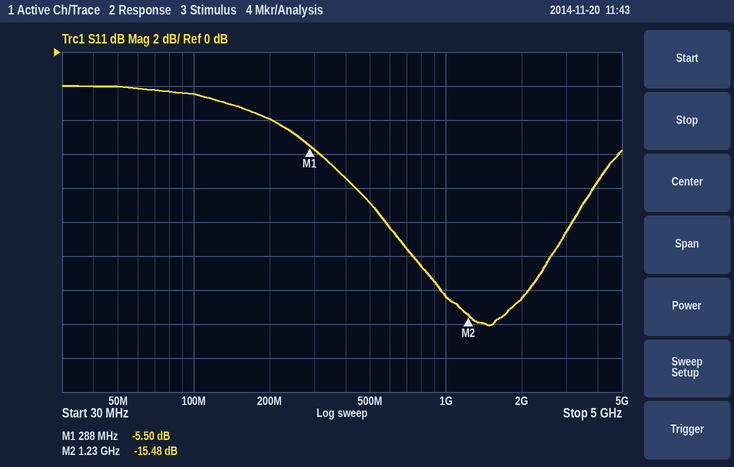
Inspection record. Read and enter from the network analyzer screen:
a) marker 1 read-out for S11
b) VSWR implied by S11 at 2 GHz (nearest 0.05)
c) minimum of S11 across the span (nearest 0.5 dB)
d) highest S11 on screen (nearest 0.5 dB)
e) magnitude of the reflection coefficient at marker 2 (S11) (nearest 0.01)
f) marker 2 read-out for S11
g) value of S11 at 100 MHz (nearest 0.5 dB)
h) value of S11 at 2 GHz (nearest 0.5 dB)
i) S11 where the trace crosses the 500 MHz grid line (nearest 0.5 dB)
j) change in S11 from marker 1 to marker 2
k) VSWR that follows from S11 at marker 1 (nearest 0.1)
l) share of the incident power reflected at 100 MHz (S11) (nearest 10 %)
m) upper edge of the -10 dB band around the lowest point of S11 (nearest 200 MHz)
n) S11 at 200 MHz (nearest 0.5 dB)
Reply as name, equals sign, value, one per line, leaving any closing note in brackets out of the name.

marker 1 read-out for S11 = -5.50 dB
VSWR implied by S11 at 2 GHz = 1.45
minimum of S11 across the span = -16.0 dB
highest S11 on screen = -2.0 dB
magnitude of the reflection coefficient at marker 2 (S11) = 0.17
marker 2 read-out for S11 = -15.48 dB
value of S11 at 100 MHz = -2.5 dB
value of S11 at 2 GHz = -14.5 dB
S11 where the trace crosses the 500 MHz grid line = -9.0 dB
change in S11 from marker 1 to marker 2 = -9.98 dB
VSWR that follows from S11 at marker 1 = 3.3
share of the incident power reflected at 100 MHz (S11) = 60 %
upper edge of the -10 dB band around the lowest point of S11 = 3.2 GHz
S11 at 200 MHz = -4.0 dB
